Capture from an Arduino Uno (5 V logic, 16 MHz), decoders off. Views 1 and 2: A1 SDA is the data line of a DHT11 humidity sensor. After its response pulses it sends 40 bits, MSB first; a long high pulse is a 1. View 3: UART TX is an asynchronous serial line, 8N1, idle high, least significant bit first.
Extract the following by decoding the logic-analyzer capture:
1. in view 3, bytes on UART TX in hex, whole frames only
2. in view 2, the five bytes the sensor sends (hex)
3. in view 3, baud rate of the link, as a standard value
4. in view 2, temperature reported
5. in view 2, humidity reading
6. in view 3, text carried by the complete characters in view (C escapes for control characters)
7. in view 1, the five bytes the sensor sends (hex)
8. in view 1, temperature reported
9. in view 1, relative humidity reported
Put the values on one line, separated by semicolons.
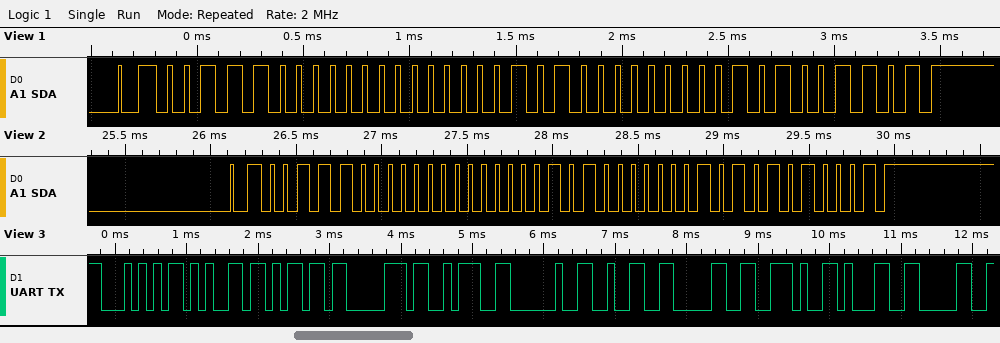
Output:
54 65 6D 70 3A 20 32 30 2E 31 30; 38 00 14 05 51; 9600 baud; 20.5 °C; 56 %; "Temp: 20.10"; 38 00 14 01 4D; 20.1 °C; 56 %
